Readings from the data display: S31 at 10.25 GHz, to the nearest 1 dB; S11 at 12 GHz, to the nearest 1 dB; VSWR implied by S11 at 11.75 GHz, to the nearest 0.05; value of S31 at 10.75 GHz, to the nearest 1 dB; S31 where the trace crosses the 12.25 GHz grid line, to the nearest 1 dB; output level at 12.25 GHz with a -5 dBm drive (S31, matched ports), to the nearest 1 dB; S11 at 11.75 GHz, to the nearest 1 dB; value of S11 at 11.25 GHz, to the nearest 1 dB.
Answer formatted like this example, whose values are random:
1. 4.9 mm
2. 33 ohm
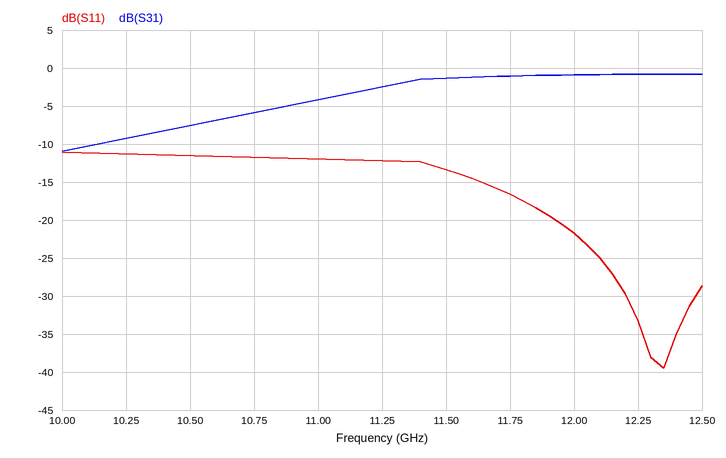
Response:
1. -9 dB
2. -22 dB
3. 1.35
4. -6 dB
5. -1 dB
6. -6 dBm
7. -17 dB
8. -12 dB
